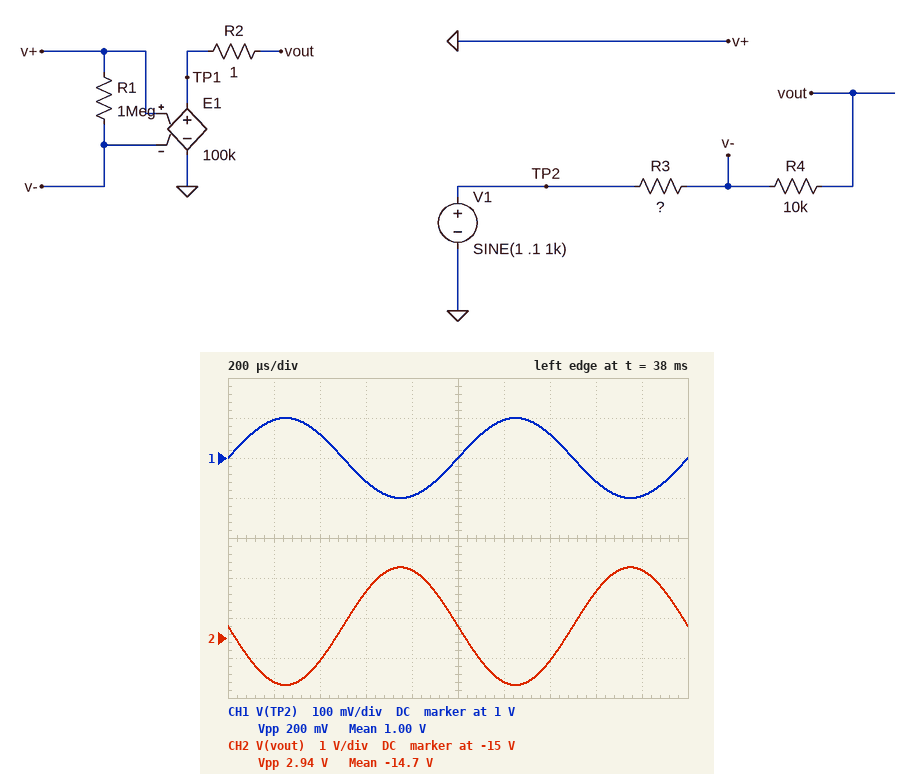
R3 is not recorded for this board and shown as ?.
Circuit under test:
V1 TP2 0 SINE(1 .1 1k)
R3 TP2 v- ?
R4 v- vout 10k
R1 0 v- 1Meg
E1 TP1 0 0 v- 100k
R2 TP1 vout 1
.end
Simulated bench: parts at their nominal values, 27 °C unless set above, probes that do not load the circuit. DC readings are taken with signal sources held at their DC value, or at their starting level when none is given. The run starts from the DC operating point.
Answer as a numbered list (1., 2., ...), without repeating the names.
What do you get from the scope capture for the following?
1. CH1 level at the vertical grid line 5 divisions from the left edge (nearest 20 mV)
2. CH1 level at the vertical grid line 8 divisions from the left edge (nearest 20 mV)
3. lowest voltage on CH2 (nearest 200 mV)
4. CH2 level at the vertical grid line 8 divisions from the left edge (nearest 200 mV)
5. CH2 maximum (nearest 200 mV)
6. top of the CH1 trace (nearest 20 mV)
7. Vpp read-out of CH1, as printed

1. 1.00 V
2. 940 mV
3. -16.2 V
4. -13.8 V
5. -13.2 V
6. 1.10 V
7. 200 mV
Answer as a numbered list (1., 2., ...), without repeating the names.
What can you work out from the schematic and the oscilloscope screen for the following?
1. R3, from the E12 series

1. 680 Ω
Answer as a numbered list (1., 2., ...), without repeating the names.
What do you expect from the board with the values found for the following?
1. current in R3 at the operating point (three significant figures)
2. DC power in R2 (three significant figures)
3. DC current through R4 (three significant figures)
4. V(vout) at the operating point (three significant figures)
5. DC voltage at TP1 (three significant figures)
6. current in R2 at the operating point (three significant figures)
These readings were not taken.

1. 1.47 mA
2. 2.16 µW
3. 1.47 mA
4. -14.7 V
5. -14.7 V
6. 1.47 mA
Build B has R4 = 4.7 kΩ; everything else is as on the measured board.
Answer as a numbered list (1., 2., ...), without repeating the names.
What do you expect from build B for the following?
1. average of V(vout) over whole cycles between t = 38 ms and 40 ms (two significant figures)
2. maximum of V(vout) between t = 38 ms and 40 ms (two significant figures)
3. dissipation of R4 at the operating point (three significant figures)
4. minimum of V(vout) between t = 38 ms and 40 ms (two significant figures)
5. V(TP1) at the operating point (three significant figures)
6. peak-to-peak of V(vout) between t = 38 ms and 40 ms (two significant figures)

1. -6.9 V
2. -6.2 V
3. 10.2 mW
4. -7.6 V
5. -6.91 V
6. 1.4 V
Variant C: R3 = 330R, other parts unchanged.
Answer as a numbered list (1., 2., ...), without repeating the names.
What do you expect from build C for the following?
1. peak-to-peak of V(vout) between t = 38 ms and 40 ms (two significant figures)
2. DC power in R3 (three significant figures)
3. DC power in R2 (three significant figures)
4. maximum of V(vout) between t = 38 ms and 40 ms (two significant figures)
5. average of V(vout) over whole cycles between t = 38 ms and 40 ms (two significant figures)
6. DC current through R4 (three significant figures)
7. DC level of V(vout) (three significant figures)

1. 6.1 V
2. 3.03 mW
3. 9.18 µW
4. -27 V
5. -30 V
6. 3.03 mA
7. -30.3 V
